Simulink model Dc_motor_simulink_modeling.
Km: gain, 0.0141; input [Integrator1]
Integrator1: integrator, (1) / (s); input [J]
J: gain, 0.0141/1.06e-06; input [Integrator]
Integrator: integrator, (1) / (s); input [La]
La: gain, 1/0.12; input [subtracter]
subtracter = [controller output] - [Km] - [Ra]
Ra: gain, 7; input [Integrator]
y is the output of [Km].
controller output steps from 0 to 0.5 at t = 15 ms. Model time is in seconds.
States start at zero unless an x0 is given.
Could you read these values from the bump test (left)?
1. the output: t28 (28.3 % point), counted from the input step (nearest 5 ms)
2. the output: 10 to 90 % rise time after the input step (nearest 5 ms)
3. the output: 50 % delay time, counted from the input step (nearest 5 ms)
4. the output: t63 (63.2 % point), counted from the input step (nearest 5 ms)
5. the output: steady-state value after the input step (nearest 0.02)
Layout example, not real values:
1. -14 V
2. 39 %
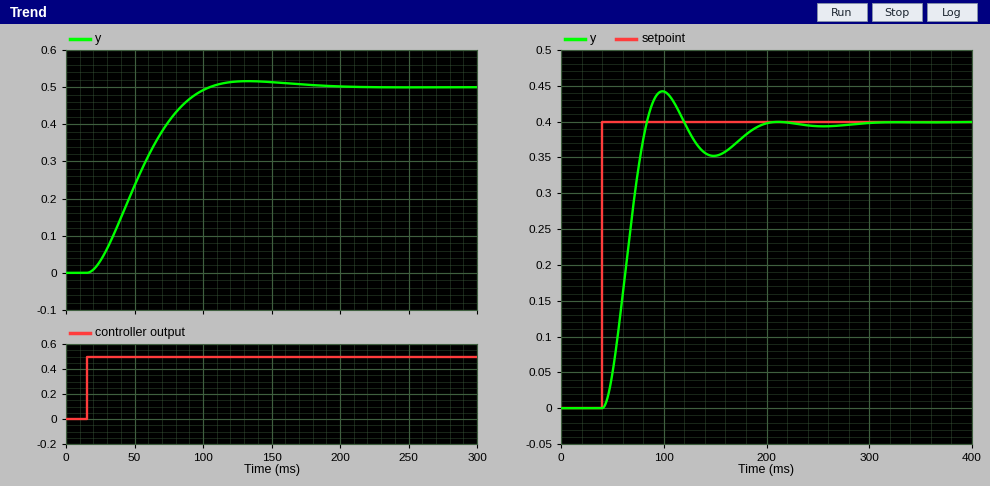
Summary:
1. 25 ms
2. 55 ms
3. 35 ms
4. 45 ms
5. 0.50
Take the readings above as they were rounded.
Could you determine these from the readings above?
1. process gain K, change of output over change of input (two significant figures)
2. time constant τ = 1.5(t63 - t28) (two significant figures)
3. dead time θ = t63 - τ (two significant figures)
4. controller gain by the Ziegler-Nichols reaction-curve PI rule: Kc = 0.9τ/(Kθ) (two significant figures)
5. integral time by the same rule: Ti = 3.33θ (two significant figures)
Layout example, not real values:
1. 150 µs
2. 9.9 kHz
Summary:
1. 1.0
2. 30 ms
3. 15 ms
4. 1.8
5. 50 ms
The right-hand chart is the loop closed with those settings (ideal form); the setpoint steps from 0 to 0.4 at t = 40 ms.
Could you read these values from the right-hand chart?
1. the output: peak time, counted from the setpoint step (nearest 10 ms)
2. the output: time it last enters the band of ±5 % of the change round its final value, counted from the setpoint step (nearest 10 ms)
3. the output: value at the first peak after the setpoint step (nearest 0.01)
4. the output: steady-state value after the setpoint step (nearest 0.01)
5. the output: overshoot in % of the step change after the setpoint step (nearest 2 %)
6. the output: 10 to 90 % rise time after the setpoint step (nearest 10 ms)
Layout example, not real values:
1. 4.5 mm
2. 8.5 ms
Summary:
1. 60 ms
2. 140 ms
3. 0.44
4. 0.40
5. 10 %
6. 30 ms
